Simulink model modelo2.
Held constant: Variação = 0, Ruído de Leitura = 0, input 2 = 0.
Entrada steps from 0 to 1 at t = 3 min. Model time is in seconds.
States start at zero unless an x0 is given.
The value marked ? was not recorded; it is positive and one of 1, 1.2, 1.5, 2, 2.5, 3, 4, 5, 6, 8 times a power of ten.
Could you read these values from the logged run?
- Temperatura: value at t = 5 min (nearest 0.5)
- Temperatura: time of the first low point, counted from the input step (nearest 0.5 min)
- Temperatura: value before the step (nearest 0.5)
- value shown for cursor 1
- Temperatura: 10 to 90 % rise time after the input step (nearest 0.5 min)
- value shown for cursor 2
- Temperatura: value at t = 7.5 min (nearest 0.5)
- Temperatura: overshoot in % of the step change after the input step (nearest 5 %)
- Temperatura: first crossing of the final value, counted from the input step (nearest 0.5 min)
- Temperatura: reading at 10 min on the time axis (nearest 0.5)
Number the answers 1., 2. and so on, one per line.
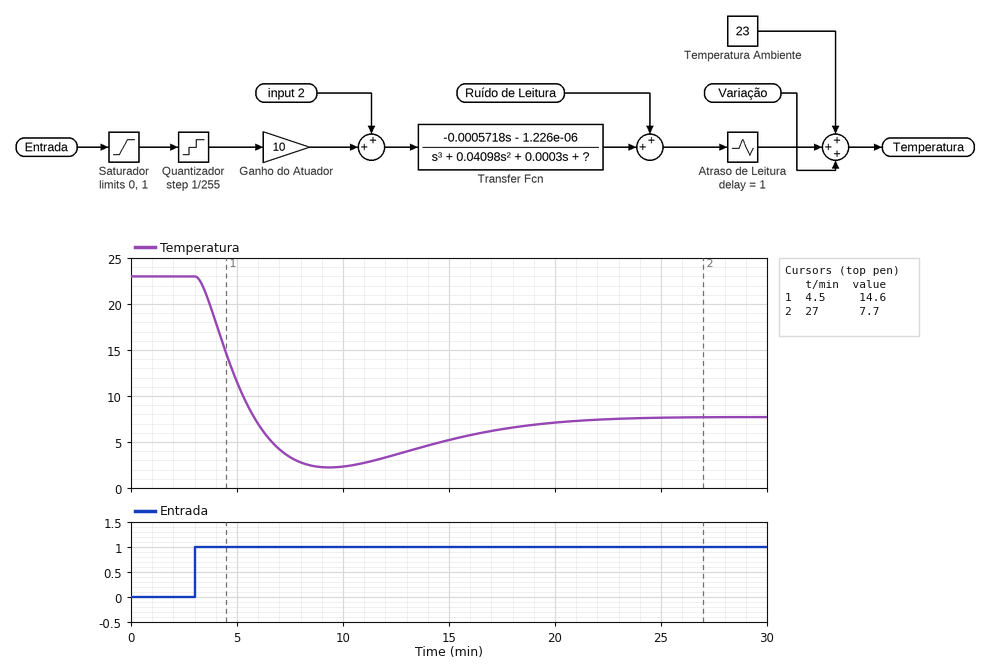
1. 11.5
2. 6.5 min
3. 23.0
4. 14.6
5. 2.0 min
6. 7.7
7. 3.5
8. 35 %
9. 3.0 min
10. 2.5
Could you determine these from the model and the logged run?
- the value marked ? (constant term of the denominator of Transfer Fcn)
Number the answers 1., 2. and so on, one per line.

1. 8e-07
